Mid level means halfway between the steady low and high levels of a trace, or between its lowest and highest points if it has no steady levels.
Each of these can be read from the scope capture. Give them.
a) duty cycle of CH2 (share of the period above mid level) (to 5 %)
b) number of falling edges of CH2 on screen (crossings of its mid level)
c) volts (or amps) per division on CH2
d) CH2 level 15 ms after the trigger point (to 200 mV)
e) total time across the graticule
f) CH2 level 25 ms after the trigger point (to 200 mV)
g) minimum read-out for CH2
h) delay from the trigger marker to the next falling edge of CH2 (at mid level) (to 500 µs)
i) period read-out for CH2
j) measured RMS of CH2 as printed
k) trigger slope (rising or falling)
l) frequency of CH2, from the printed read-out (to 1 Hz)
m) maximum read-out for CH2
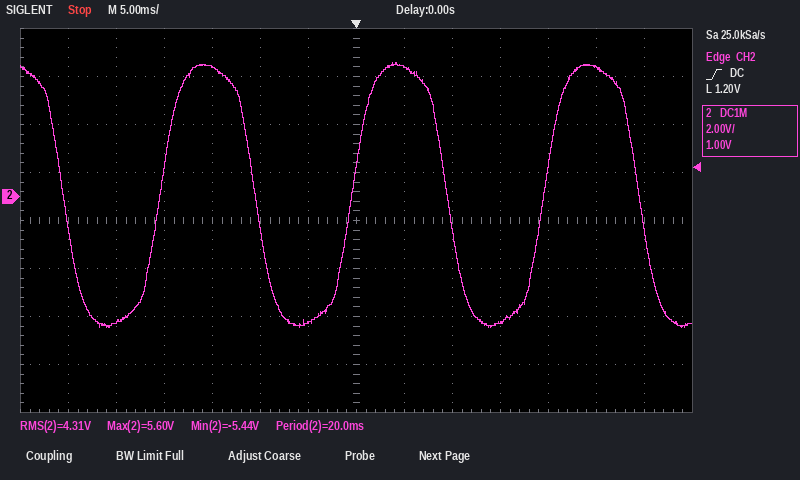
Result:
50 %
4
2 V
-5.2 V
70 ms
5.4 V
-5.44 V
9.5 ms
20.0 ms
4.31 V
rising
50 Hz
5.60 V
